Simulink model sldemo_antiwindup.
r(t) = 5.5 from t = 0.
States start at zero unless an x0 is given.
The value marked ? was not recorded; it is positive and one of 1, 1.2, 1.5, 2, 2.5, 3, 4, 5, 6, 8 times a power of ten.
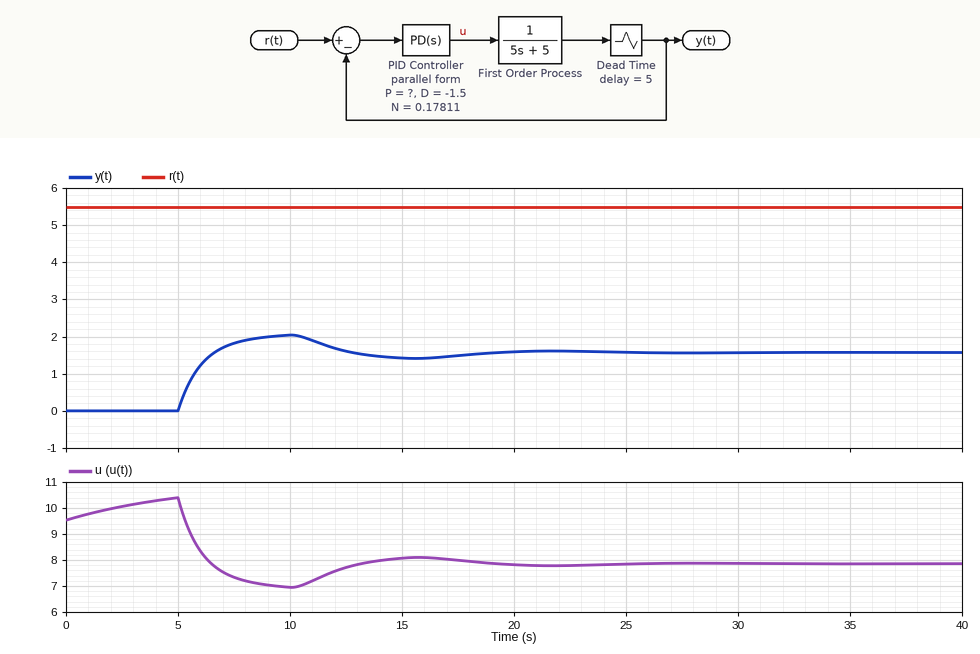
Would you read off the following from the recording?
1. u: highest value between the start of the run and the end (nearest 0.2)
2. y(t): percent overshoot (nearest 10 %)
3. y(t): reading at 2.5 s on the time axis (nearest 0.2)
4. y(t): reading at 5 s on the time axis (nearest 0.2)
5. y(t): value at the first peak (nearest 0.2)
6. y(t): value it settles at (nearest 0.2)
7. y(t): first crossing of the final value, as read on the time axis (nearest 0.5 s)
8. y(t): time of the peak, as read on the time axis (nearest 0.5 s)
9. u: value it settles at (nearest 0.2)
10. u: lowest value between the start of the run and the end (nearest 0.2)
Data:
10.4
30 %
0.0
0.0
2.0
1.6
6.5 s
10.0 s
7.8
7.0
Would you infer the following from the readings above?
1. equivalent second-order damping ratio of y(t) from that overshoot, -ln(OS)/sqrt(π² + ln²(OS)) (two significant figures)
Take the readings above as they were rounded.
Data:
0.36
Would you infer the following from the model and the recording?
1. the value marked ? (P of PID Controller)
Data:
2
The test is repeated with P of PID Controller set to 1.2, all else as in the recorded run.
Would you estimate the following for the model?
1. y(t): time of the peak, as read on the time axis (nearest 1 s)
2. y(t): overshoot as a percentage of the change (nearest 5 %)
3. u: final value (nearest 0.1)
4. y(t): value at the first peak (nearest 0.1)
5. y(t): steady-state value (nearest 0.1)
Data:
10 s
10 %
5.3
1.2
1.1
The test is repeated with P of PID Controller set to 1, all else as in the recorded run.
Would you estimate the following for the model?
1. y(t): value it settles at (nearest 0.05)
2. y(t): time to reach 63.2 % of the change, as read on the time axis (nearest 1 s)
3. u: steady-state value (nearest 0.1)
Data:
0.90
6 s
4.6
